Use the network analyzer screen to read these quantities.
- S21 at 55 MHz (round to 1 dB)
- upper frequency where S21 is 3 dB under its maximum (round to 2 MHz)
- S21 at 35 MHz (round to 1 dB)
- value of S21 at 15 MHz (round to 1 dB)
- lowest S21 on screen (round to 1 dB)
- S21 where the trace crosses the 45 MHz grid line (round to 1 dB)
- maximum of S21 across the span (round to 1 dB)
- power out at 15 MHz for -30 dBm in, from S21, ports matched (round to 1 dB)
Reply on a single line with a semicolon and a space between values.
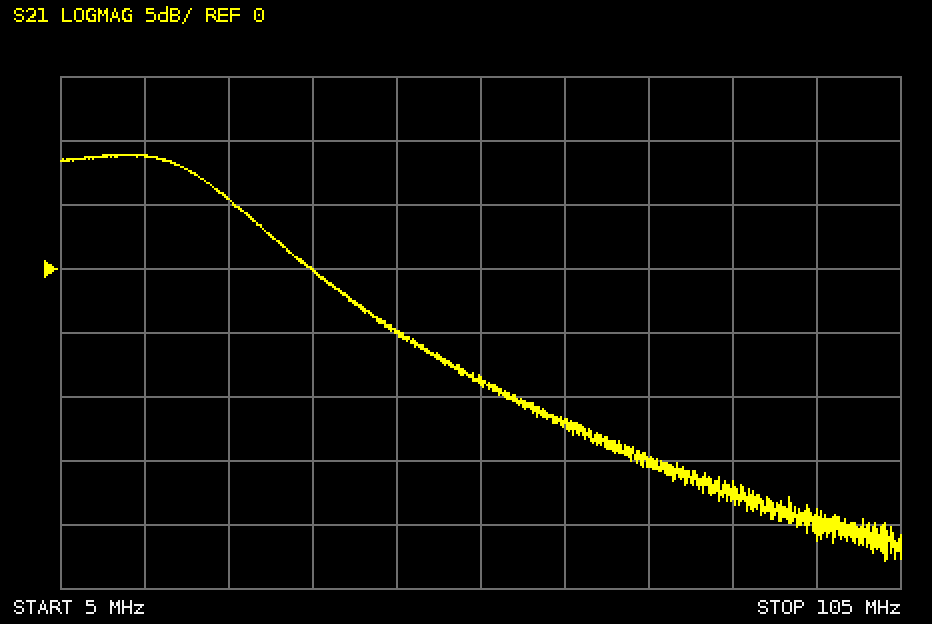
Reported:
-9 dB; 24 MHz; 0 dB; 9 dB; -23 dB; -5 dB; 9 dB; -21 dBm
